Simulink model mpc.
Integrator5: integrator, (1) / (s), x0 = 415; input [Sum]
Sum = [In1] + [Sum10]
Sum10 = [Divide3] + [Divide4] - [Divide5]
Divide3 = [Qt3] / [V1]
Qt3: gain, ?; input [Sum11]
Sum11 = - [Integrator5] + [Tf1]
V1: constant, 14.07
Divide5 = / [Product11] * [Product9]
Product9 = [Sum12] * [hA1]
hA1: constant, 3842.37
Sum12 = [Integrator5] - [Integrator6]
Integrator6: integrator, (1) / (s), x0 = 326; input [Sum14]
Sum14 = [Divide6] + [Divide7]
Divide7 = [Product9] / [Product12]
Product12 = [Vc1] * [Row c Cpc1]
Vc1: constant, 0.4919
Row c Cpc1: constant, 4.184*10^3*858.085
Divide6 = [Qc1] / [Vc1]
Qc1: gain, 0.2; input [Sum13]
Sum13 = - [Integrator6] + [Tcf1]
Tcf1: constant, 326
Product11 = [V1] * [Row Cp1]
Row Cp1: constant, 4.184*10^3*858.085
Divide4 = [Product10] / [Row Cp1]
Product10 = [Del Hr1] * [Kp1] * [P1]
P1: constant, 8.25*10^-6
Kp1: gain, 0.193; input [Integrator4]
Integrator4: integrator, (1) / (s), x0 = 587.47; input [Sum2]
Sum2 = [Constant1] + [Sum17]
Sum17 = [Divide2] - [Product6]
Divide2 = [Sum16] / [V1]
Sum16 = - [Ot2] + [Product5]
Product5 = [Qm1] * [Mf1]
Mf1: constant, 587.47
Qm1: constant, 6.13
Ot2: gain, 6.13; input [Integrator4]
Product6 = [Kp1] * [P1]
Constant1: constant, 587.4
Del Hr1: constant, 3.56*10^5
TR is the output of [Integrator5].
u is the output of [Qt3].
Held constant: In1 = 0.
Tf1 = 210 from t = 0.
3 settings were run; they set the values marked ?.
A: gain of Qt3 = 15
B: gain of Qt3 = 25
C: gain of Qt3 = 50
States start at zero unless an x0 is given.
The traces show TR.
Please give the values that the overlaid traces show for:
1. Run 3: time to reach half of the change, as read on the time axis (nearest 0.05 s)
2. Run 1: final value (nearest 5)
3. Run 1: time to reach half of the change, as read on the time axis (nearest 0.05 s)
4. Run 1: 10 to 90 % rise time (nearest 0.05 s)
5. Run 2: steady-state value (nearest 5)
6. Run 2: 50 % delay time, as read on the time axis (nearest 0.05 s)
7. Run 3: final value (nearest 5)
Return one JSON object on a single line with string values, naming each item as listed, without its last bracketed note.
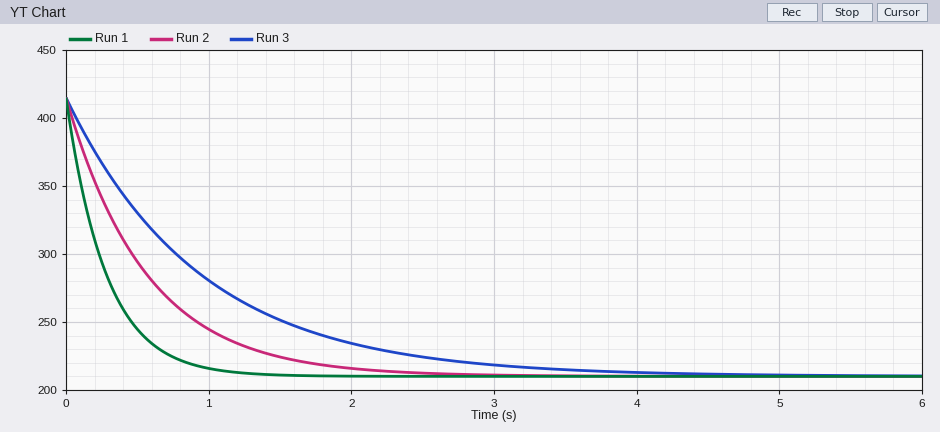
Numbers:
{"Run 3: time to reach half of the change, as read on the time axis": "0.65 s", "Run 1: final value": "210", "Run 1: time to reach half of the change, as read on the time axis": "0.20 s", "Run 1: 10 to 90 % rise time": "0.60 s", "Run 2: steady-state value": "210", "Run 2: 50 % delay time, as read on the time axis": "0.40 s", "Run 3: final value": "210"}
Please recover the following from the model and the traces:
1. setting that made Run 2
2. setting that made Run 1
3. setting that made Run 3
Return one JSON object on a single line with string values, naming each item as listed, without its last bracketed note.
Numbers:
{"setting that made Run 2": "B", "setting that made Run 1": "C", "setting that made Run 3": "A"}
